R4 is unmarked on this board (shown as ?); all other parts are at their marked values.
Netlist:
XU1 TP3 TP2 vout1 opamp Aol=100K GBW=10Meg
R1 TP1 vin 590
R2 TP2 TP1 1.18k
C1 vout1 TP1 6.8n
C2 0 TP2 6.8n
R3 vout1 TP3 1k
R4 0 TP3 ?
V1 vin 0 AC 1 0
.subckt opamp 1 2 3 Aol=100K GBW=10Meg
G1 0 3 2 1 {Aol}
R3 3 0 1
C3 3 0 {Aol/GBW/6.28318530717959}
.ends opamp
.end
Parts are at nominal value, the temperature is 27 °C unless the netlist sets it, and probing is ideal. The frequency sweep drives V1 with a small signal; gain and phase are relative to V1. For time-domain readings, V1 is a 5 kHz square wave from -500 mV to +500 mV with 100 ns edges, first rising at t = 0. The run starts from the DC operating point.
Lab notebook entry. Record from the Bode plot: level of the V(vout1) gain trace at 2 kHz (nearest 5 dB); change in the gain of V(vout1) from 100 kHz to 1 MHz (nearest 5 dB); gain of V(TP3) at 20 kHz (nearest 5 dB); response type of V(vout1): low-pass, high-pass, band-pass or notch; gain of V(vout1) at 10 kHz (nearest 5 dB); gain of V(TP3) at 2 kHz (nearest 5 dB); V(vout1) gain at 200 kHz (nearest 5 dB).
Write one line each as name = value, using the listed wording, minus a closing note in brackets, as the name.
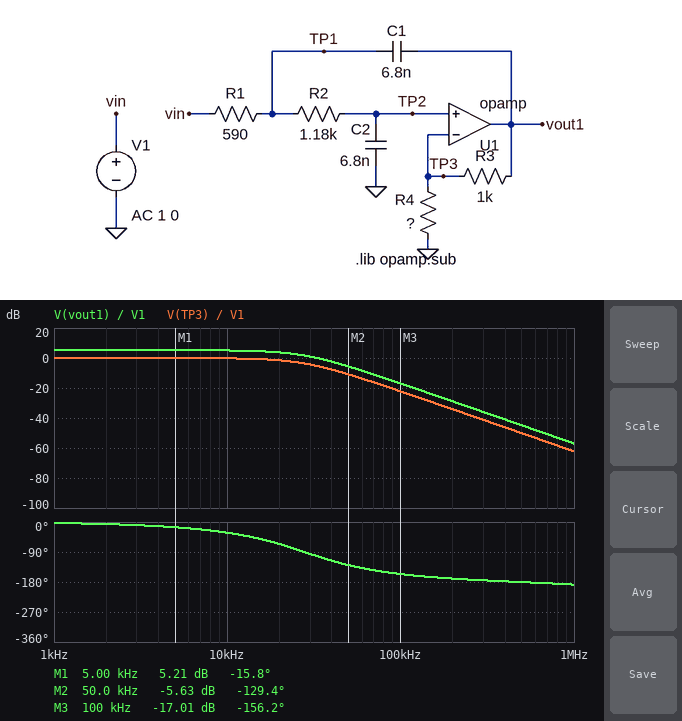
level of the V(vout1) gain trace at 2 kHz = 5 dB
change in the gain of V(vout1) from 100 kHz to 1 MHz = -40 dB
gain of V(TP3) at 20 kHz = 0 dB
response type of V(vout1): low-pass, high-pass, band-pass or notch = low-pass
gain of V(vout1) at 10 kHz = 5 dB
gain of V(TP3) at 2 kHz = 0 dB
V(vout1) gain at 200 kHz = -30 dB
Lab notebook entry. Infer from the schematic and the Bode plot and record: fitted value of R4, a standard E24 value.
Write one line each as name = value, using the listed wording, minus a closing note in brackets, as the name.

fitted value of R4, a standard E24 value = 1.2 kΩ
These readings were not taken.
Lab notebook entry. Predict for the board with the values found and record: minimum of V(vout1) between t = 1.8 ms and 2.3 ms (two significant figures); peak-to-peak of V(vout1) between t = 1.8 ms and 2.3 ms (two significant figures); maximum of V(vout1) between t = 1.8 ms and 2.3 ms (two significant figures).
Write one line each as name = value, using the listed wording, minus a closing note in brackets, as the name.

minimum of V(vout1) between t = 1.8 ms and 2.3 ms = -960 mV
peak-to-peak of V(vout1) between t = 1.8 ms and 2.3 ms = 1.9 V
maximum of V(vout1) between t = 1.8 ms and 2.3 ms = 960 mV
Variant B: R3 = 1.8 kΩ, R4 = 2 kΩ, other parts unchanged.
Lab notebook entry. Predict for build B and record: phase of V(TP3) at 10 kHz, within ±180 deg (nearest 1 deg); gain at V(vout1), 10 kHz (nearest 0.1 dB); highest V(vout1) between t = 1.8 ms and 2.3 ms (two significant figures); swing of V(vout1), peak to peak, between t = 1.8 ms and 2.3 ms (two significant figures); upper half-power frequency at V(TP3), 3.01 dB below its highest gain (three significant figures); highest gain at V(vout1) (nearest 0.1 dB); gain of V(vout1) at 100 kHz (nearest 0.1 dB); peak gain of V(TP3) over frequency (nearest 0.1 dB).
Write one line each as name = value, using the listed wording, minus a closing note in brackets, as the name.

phase of V(TP3) at 10 kHz, within ±180 deg = -31 deg
gain at V(vout1), 10 kHz = 5.4 dB
highest V(vout1) between t = 1.8 ms and 2.3 ms = 1.0 V
swing of V(vout1), peak to peak, between t = 1.8 ms and 2.3 ms = 2.0 V
upper half-power frequency at V(TP3), 3.01 dB below its highest gain = 26.7 kHz
highest gain at V(vout1) = 5.6 dB
gain of V(vout1) at 100 kHz = -16.7 dB
peak gain of V(TP3) over frequency = 0 dB
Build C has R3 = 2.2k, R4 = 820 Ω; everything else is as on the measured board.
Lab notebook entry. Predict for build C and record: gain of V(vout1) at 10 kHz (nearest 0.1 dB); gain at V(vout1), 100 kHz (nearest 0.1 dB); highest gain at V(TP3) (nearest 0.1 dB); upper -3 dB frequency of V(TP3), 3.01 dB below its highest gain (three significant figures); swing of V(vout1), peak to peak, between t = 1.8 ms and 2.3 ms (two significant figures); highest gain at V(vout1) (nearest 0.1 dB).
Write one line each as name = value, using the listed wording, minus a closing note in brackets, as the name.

gain of V(vout1) at 10 kHz = 12.5 dB
gain at V(vout1), 100 kHz = -10.3 dB
highest gain at V(TP3) = 13.1 dB
upper -3 dB frequency of V(TP3), 3.01 dB below its highest gain = 30.3 kHz
swing of V(vout1), peak to peak, between t = 1.8 ms and 2.3 ms = 8.9 V
highest gain at V(vout1) = 24.5 dB
